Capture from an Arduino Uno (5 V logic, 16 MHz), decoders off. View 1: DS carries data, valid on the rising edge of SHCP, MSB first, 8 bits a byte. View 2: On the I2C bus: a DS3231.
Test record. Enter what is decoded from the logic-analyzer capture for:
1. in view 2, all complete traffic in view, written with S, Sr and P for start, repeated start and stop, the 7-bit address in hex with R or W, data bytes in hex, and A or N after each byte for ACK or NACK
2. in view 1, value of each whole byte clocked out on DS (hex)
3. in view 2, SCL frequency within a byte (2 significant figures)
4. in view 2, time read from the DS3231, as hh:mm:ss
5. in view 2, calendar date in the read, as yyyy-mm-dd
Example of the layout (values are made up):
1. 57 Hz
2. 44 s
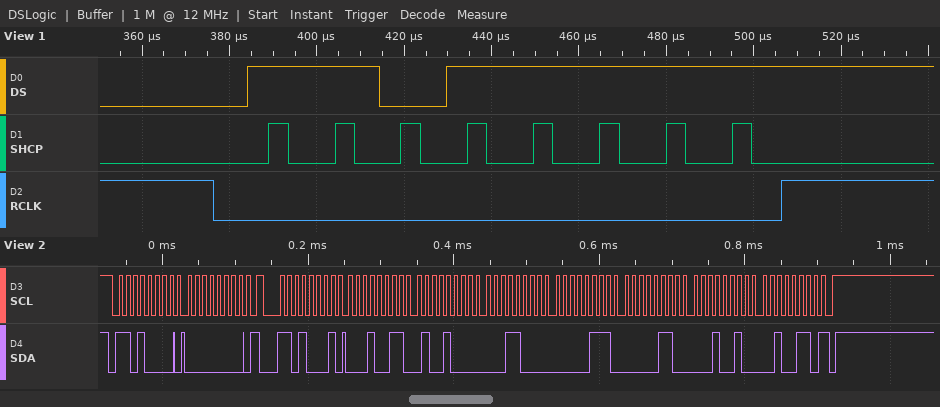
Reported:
1. S 68W A 00 A Sr 68R A 13 A 48 A 18 A 07 A 06 A 12 A 26 N P
2. 0xDF
3. 100 kHz
4. 18:48:13
5. 2026-12-06
